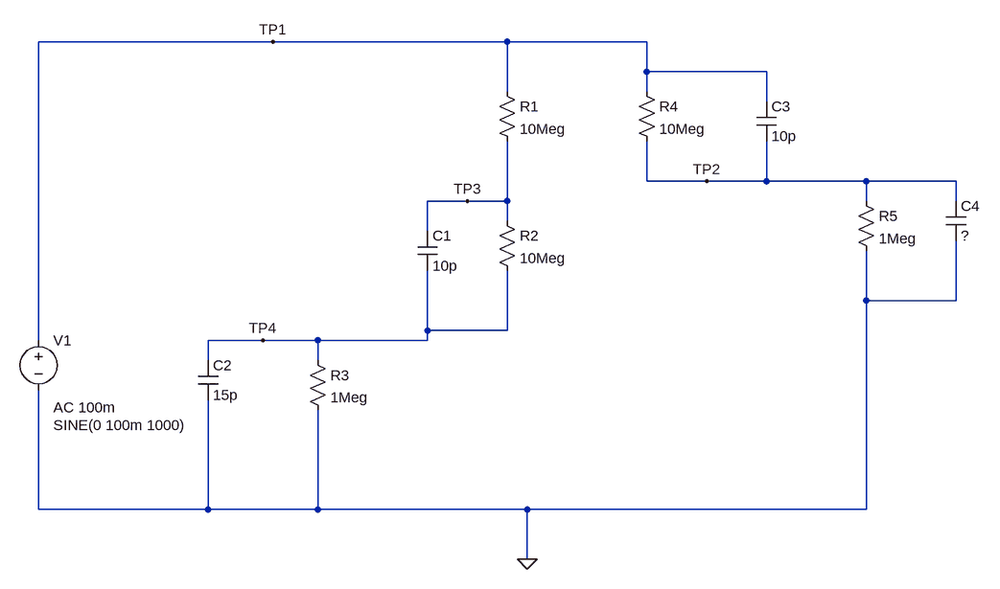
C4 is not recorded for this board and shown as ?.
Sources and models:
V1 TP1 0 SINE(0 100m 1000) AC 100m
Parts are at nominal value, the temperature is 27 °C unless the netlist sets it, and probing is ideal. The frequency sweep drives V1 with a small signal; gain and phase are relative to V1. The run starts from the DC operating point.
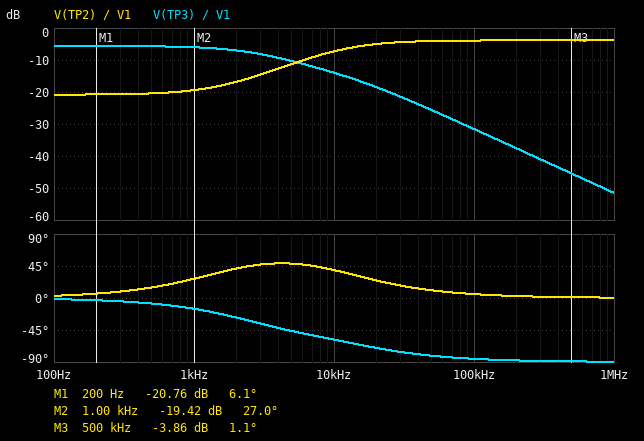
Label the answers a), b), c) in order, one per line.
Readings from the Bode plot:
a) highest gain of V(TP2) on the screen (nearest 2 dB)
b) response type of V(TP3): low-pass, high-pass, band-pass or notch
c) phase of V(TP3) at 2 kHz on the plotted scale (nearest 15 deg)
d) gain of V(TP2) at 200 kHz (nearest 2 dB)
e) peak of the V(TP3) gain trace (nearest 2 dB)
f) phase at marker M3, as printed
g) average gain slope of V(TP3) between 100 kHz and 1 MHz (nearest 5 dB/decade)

a) -4 dB
b) low-pass
c) -30 deg
d) -4 dB
e) -6 dB
f) 1.1 deg
g) -20 dB/decade
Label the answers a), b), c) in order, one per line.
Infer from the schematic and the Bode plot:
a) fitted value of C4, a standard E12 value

a) 5.6 pF
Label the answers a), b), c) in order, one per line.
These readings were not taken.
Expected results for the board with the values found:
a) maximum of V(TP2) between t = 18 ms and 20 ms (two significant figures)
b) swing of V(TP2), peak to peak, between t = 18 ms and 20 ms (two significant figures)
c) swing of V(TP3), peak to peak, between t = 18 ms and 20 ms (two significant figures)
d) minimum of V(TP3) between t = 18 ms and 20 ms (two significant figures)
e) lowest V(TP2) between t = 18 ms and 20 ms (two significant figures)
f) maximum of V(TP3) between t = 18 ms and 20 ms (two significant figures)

a) 11 mV
b) 21 mV
c) 100 mV
d) -50 mV
e) -11 mV
f) 50 mV
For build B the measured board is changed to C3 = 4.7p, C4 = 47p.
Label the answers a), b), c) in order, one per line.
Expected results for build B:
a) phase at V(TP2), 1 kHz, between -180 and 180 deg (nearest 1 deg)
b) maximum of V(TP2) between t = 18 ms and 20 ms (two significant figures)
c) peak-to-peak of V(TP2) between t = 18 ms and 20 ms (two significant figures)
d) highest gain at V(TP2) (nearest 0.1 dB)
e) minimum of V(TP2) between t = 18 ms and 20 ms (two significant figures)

a) 0 deg
b) 9.1 mV
c) 18 mV
d) -20.8 dB
e) -9.1 mV
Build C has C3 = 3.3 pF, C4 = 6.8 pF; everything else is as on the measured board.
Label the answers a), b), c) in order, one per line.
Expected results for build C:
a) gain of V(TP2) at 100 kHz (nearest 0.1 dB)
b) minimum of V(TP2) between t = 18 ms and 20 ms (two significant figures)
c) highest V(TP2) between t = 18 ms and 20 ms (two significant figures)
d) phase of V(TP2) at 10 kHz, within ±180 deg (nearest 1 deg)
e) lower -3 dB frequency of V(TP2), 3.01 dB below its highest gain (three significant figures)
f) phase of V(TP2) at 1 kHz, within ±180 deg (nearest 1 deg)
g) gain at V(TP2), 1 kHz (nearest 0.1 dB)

a) -9.8 dB
b) -9.3 mV
c) 9.3 mV
d) 34 deg
e) 15.9 kHz
f) 8 deg
g) -20.7 dB
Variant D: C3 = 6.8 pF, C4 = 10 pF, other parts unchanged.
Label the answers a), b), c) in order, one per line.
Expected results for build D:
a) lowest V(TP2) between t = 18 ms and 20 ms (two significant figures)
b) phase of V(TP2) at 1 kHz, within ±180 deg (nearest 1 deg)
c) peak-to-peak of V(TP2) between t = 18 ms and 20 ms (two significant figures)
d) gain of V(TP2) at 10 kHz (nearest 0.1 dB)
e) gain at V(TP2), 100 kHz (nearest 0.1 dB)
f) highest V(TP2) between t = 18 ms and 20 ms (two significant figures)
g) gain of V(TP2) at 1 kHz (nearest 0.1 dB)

a) -9.8 mV
b) 18 deg
c) 20 mV
d) -10.8 dB
e) -7.9 dB
f) 9.8 mV
g) -20.1 dB
